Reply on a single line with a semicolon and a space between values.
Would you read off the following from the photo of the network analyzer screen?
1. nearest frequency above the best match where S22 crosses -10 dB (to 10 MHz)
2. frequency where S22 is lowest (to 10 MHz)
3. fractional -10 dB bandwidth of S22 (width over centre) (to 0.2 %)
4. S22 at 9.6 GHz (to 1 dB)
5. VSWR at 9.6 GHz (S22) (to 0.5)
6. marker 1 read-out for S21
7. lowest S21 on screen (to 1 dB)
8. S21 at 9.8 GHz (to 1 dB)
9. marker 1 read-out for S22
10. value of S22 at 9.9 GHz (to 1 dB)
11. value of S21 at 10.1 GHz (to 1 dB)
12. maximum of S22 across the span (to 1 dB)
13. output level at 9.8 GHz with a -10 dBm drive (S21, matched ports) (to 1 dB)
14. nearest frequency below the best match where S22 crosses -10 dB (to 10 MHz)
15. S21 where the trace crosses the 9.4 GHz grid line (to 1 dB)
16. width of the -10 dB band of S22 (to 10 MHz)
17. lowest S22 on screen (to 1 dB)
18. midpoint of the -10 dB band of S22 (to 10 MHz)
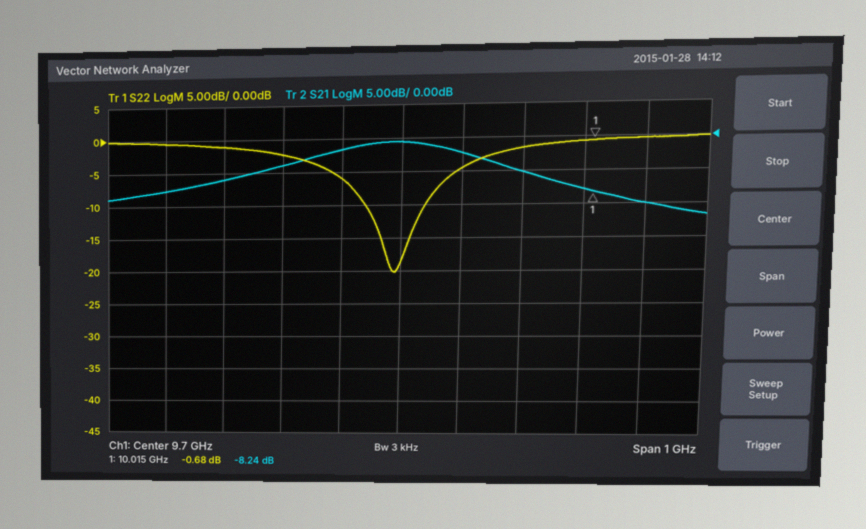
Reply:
9.74 GHz; 9.69 GHz; 1.0 %; -6 dB; 3.0; -8.24 dB; -12 dB; -2 dB; -0.68 dB; -2 dB; -10 dB; 0 dB; -12 dBm; 9.64 GHz; -6 dB; 100 MHz; -20 dB; 9.69 GHz
